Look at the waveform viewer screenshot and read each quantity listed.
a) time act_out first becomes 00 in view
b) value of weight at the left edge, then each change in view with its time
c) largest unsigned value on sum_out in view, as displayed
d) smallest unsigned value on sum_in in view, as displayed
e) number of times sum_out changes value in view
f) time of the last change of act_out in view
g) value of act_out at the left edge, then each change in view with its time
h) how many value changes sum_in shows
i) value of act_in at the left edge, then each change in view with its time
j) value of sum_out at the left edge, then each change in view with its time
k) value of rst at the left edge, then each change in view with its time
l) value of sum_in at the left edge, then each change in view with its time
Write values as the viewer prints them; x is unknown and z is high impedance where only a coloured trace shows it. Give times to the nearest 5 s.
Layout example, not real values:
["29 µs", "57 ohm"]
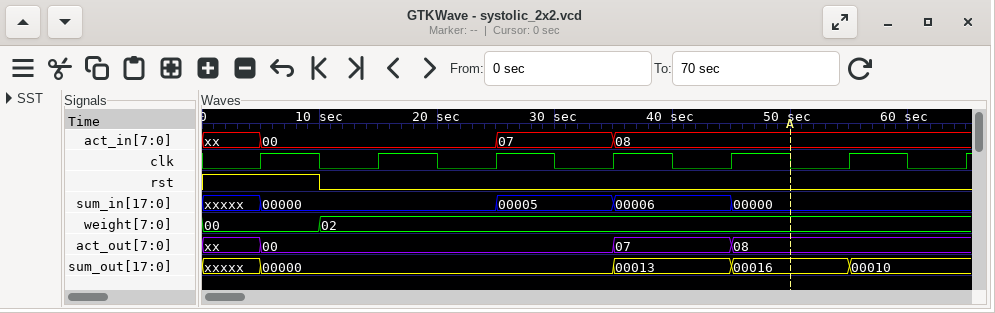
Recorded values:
["5 s", "00, 02 at 10 s", "00016", "00000", "4", "45 s", "xx, 00 at 5 s, 07 at 35 s, 08 at 45 s", "4", "xx, 00 at 5 s, 07 at 25 s, 08 at 35 s", "xxxxx, 00000 at 5 s, 00013 at 35 s, 00016 at 45 s, 00010 at 55 s", "1, 0 at 10 s", "xxxxx, 00000 at 5 s, 00005 at 25 s, 00006 at 35 s, 00000 at 45 s"]
